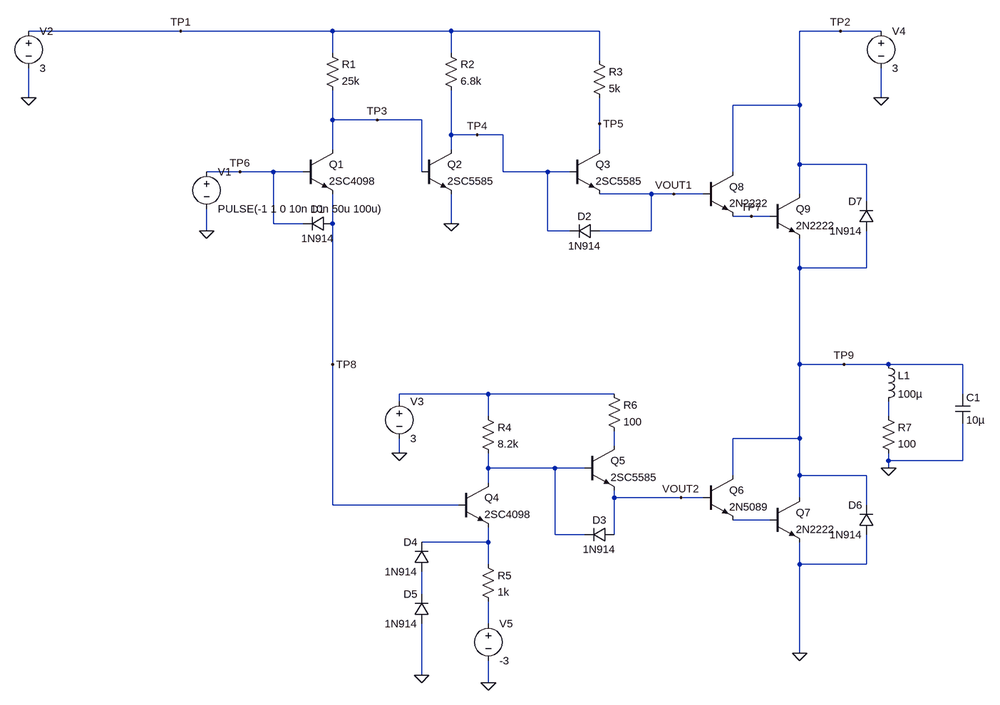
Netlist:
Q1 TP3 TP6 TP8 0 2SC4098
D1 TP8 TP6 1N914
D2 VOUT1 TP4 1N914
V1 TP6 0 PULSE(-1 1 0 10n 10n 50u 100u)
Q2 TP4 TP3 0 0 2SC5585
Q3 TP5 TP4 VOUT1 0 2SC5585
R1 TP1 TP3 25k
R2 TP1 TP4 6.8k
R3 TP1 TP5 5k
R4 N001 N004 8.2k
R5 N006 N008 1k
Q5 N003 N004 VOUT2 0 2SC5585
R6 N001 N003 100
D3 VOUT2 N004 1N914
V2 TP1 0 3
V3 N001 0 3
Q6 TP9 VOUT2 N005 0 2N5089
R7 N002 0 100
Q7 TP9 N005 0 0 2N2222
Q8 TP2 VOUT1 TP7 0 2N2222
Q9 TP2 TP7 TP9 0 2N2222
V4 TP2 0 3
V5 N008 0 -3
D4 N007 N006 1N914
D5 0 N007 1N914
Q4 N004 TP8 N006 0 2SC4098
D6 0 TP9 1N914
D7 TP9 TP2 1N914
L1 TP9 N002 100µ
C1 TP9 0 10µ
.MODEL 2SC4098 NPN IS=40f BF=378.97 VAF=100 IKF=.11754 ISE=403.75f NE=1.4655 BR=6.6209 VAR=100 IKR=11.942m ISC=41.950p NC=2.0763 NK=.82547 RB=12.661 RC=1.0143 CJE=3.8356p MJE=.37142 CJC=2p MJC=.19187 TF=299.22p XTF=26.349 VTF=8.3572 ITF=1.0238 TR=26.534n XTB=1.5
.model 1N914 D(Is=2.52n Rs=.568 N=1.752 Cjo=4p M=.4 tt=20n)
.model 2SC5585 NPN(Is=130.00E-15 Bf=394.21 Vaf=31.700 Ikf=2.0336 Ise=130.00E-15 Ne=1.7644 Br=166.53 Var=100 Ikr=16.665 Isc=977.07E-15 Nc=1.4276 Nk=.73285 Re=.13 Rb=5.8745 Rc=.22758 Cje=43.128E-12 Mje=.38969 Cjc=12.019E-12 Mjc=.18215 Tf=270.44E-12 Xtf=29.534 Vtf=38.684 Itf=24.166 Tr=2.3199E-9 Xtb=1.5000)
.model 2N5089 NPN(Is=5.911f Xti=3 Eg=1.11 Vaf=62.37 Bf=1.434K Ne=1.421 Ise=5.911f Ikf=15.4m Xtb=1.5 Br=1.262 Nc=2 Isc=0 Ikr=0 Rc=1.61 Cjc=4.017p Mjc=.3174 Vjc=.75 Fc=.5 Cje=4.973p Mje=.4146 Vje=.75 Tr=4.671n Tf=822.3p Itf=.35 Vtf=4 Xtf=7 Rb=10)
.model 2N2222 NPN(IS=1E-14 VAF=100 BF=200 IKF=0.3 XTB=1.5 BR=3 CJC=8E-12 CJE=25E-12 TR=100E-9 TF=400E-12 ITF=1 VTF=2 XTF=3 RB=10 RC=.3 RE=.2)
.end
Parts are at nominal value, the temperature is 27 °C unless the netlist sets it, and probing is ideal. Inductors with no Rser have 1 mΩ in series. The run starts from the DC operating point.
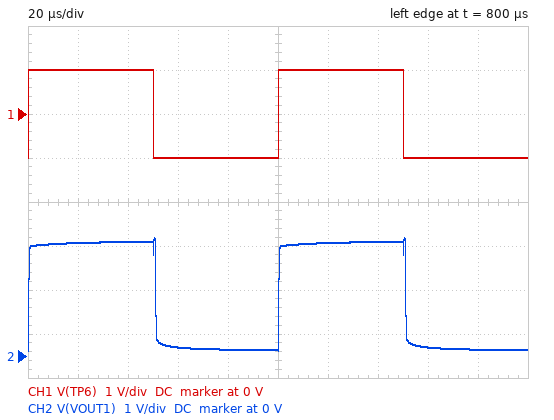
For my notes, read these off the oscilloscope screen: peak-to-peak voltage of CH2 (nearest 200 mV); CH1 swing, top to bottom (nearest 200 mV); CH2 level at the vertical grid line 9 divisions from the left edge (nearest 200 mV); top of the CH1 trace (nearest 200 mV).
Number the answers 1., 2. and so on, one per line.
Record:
1. 2.6 V
2. 2.0 V
3. 200 mV
4. 1.0 V
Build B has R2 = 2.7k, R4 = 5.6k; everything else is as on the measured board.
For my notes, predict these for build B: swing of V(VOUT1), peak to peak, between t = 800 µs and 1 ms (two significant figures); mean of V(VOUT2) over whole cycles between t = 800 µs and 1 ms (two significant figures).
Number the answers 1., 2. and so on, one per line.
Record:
1. 2.5 V
2. 630 mV
